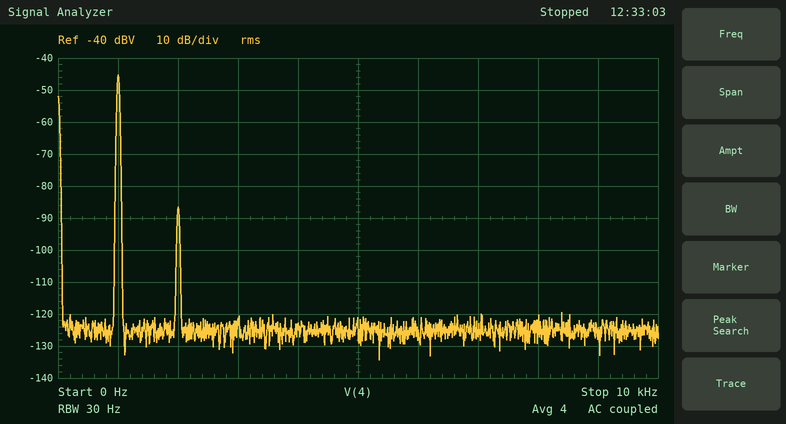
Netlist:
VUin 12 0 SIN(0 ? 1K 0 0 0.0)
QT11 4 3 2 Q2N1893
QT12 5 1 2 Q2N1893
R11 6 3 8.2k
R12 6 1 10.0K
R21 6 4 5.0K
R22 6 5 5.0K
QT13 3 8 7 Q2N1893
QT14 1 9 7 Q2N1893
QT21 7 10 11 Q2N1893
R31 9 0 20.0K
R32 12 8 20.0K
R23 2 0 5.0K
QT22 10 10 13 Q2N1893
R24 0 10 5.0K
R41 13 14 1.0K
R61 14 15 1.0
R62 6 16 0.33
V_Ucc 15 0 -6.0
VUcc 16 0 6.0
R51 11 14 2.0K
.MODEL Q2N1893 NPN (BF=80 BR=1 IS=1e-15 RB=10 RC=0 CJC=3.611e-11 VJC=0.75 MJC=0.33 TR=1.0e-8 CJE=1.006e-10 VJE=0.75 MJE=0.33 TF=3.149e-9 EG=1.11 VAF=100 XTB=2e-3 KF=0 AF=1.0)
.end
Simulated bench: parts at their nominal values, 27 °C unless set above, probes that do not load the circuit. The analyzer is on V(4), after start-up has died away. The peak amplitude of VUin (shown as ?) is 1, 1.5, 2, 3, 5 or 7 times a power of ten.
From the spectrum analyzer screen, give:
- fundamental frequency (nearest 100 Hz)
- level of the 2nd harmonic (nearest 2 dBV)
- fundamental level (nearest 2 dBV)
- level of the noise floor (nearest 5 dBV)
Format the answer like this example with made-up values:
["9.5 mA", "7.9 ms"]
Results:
["1.0 kHz", "-86 dBV", "-46 dBV", "-125 dBV"]
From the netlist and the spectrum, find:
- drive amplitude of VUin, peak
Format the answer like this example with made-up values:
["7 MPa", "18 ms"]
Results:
["700 µV"]
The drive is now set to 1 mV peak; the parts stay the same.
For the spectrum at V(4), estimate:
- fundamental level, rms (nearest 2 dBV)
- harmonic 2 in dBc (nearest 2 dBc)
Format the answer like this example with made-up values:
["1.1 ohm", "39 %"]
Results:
["-42 dBV", "-38 dBc"]
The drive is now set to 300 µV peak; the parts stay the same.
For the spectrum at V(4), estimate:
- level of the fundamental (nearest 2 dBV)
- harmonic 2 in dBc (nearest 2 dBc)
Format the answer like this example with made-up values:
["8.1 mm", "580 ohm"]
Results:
["-52 dBV", "-48 dBc"]
